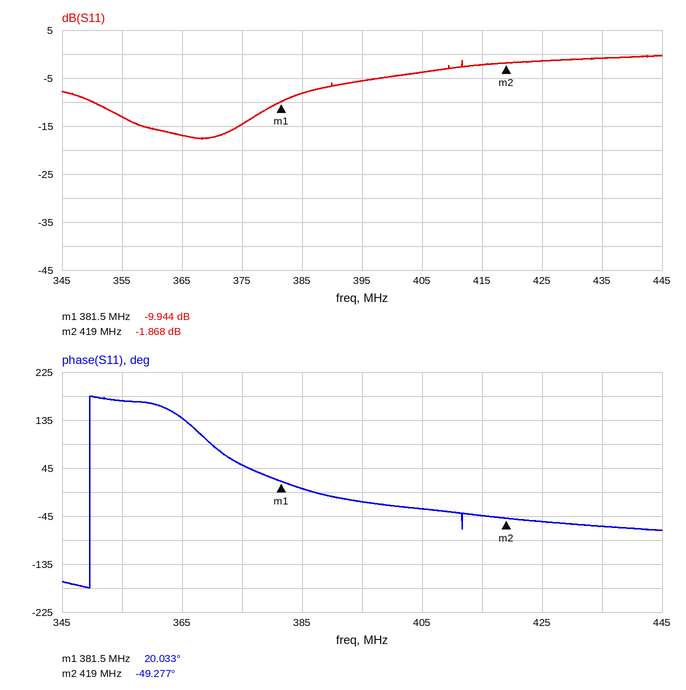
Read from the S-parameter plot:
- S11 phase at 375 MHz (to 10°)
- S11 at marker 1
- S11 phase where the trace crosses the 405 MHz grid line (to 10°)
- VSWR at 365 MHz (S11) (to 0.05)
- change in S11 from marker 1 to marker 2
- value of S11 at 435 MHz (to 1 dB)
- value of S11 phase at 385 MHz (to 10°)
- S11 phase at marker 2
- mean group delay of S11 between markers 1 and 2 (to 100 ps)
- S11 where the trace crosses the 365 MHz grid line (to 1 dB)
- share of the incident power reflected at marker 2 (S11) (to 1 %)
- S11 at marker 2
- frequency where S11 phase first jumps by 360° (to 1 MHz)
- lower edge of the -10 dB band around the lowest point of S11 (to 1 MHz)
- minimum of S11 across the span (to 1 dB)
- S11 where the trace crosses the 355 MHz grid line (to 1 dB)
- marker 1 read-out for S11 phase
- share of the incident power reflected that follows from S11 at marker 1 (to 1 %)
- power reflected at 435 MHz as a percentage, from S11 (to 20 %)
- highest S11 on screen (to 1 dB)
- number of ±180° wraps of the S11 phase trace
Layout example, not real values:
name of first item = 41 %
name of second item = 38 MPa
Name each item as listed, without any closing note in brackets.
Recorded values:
S11 phase at 375 MHz = 50°
S11 at marker 1 = -9.944 dB
S11 phase where the trace crosses the 405 MHz grid line = -30°
VSWR at 365 MHz (S11) = 1.35
change in S11 from marker 1 to marker 2 = 8.076 dB
value of S11 at 435 MHz = -1 dB
value of S11 phase at 385 MHz = 10°
S11 phase at marker 2 = -49.277°
mean group delay of S11 between markers 1 and 2 = 5.1 ns
S11 where the trace crosses the 365 MHz grid line = -17 dB
share of the incident power reflected at marker 2 (S11) = 65 %
S11 at marker 2 = -1.868 dB
frequency where S11 phase first jumps by 360° = 350 MHz
lower edge of the -10 dB band around the lowest point of S11 = 350 MHz
minimum of S11 across the span = -18 dB
S11 where the trace crosses the 355 MHz grid line = -13 dB
marker 1 read-out for S11 phase = 20.033°
share of the incident power reflected that follows from S11 at marker 1 = 10 %
power reflected at 435 MHz as a percentage, from S11 = 80 %
highest S11 on screen = 0 dB
number of ±180° wraps of the S11 phase trace = 1
